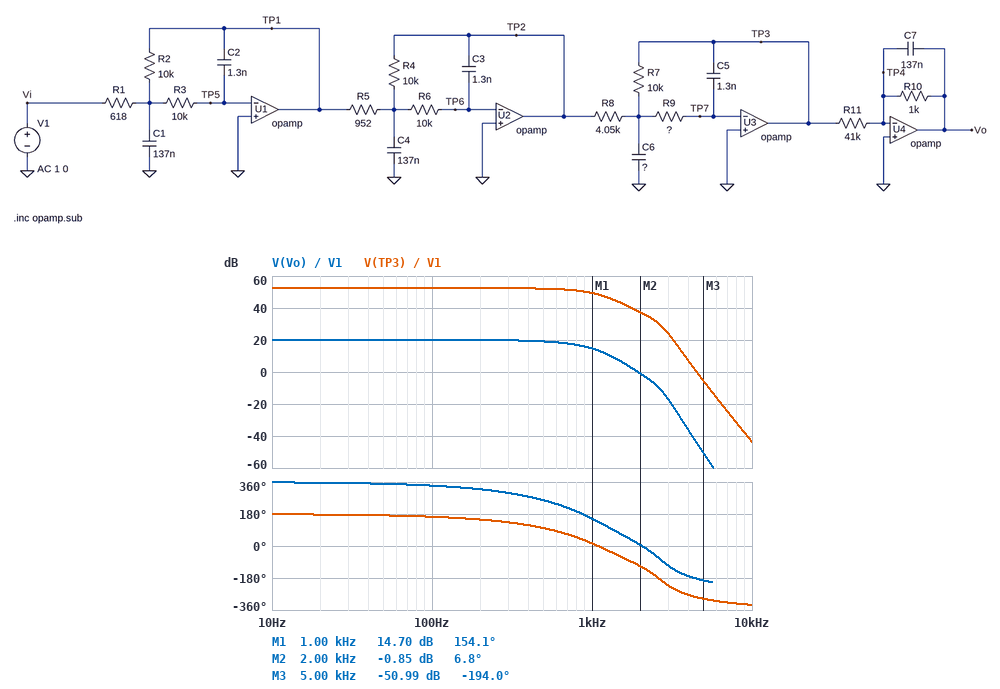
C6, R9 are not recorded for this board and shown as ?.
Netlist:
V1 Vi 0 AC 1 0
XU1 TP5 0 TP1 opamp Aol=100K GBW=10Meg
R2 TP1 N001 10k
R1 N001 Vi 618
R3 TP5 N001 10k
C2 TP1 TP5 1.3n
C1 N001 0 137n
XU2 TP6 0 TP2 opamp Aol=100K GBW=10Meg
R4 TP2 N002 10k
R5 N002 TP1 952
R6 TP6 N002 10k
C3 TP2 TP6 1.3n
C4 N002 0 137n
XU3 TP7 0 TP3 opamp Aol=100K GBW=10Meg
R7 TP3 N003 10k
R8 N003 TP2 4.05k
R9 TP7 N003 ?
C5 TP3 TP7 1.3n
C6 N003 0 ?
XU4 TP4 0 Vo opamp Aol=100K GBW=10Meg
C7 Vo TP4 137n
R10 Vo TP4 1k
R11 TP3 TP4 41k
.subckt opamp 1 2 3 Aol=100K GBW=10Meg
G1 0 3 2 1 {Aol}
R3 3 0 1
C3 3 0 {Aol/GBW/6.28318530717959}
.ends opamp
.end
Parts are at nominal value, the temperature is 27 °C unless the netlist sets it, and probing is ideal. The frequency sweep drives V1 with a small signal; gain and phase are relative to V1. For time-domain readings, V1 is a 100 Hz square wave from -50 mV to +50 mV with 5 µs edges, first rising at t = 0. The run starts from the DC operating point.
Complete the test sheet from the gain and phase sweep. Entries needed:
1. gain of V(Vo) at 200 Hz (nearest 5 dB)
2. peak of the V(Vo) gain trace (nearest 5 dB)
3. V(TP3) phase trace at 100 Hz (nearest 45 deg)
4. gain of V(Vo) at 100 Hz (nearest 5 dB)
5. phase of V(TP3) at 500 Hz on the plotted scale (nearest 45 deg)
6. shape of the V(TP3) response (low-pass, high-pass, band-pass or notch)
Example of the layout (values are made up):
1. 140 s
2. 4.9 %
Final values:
1. 20 dB
2. 20 dB
3. 180 deg
4. 20 dB
5. 90 deg
6. low-pass
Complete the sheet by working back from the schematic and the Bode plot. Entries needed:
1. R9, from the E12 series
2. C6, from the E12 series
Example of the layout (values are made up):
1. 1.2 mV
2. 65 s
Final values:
1. 3.9 kΩ
2. 68 nF
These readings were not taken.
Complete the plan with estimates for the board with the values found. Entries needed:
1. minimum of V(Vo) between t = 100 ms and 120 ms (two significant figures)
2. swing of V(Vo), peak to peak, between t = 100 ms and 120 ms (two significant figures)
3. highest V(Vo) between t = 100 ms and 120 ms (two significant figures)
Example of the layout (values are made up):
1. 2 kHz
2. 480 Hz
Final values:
1. -530 mV
2. 1.1 V
3. 530 mV
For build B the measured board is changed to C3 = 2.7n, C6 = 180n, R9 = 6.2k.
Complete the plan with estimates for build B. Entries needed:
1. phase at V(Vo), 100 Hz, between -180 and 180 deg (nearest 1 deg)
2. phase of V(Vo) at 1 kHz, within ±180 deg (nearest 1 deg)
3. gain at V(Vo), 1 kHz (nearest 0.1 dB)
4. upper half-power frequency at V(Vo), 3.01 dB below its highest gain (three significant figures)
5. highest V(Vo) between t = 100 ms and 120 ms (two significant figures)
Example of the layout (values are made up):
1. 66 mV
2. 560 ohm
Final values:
1. -27 deg
2. 107 deg
3. 13.5 dB
4. 585 Hz
5. 530 mV
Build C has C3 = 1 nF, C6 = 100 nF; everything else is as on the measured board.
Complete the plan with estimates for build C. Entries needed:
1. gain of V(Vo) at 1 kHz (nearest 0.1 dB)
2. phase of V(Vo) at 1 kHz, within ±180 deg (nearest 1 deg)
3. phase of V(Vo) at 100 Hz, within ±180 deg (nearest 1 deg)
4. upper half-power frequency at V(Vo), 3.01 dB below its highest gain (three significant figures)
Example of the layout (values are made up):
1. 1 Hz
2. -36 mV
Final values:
1. 16.7 dB
2. 167 deg
3. -19 deg
4. 936 Hz
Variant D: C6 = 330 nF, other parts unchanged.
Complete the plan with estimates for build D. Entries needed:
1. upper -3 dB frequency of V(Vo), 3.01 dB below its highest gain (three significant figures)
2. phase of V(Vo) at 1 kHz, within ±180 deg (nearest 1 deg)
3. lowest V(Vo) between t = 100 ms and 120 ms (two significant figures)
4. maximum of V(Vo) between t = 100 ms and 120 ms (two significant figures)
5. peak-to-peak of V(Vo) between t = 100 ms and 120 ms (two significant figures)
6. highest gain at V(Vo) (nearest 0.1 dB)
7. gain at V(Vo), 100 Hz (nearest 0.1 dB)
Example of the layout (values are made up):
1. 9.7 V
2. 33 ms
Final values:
1. 1.29 kHz
2. 137 deg
3. -730 mV
4. 730 mV
5. 1.5 V
6. 23.1 dB
7. 20.2 dB
